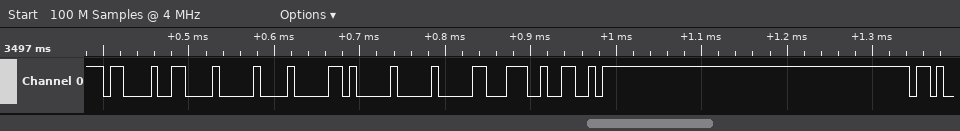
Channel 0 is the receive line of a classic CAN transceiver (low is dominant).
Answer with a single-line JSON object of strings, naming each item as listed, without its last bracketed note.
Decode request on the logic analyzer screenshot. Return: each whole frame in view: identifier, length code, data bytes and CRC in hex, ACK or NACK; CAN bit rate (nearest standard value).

{"each whole frame in view: identifier, length code, data bytes and CRC in hex, ACK or NACK": "ID 613, DLC 4, data 01 05 00 01, CRC 0E4C, ACK", "CAN bit rate": "125 kbit/s"}
